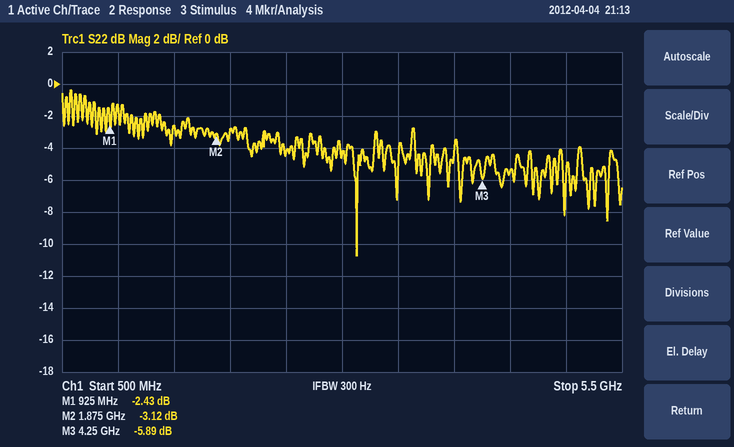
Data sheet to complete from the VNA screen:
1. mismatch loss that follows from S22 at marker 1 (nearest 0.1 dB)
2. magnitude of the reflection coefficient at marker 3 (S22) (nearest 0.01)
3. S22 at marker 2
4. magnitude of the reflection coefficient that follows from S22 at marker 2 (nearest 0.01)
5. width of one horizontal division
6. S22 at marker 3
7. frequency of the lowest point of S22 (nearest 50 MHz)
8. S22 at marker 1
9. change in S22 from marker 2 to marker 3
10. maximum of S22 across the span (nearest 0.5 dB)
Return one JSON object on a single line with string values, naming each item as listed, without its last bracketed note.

{"mismatch loss that follows from S22 at marker 1": "3.7 dB", "magnitude of the reflection coefficient at marker 3 (S22)": "0.51", "S22 at marker 2": "-3.12 dB", "magnitude of the reflection coefficient that follows from S22 at marker 2": "0.70", "width of one horizontal division": "500 MHz", "S22 at marker 3": "-5.89 dB", "frequency of the lowest point of S22": "3.15 GHz", "S22 at marker 1": "-2.43 dB", "change in S22 from marker 2 to marker 3": "-2.77 dB", "maximum of S22 across the span": "-0.5 dB"}
